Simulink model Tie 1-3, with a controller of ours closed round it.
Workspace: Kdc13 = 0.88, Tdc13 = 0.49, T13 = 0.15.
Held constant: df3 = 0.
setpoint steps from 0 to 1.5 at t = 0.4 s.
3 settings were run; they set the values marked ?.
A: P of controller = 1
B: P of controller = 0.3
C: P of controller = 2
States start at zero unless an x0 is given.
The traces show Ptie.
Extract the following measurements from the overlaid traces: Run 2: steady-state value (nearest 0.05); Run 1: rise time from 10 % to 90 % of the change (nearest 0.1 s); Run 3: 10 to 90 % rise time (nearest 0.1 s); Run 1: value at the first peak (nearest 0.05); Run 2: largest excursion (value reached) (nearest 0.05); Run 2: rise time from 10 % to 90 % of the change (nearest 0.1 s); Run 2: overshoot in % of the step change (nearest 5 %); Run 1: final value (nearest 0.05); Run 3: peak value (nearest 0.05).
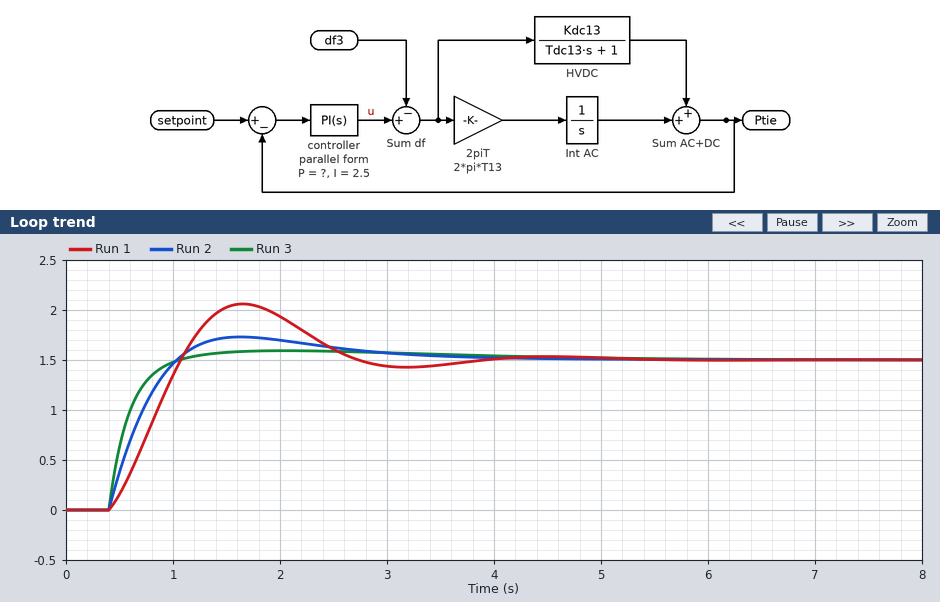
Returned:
1.50
0.5 s
0.4 s
2.05
1.75
0.5 s
15 %
1.50
1.60
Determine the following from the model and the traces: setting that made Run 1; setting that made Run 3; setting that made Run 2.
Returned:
B
C
A
